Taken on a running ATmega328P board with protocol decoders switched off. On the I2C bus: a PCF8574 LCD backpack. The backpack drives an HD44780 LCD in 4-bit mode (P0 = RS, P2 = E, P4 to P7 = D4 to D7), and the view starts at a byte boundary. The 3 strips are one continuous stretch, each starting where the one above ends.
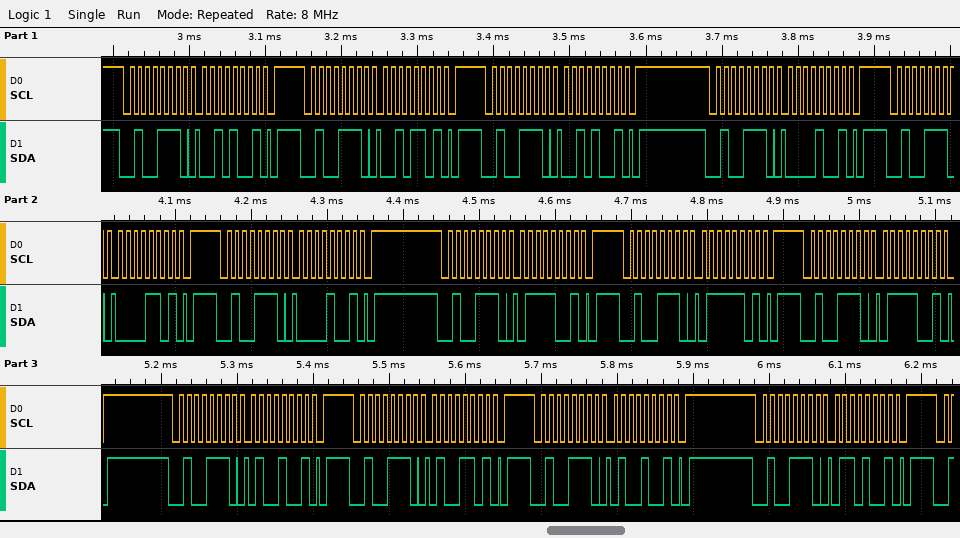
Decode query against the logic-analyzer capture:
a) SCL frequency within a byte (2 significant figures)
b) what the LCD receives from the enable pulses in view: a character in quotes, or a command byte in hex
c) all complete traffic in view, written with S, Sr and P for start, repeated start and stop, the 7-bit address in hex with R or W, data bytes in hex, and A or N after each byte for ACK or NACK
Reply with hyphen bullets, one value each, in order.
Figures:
- 100 kHz
- ' ' 't'
- S 27W A 29 A P S 27W A 2D A P S 27W A 29 A P S 27W A 09 A P S 27W A 0D A P S 27W A 09 A P S 27W A 79 A P S 27W A 7D A P S 27W A 79 A P S 27W A 49 A P S 27W A 4D A P S 27W A 49 A P S 27W A 69 A P
